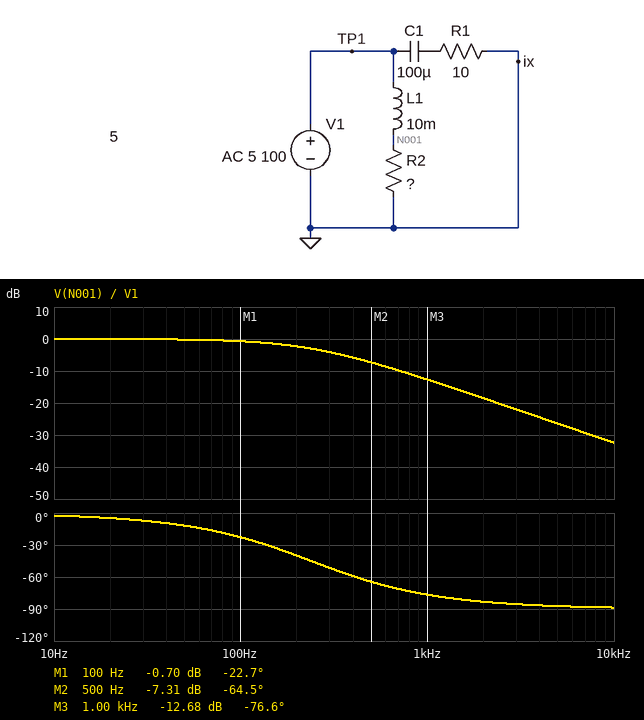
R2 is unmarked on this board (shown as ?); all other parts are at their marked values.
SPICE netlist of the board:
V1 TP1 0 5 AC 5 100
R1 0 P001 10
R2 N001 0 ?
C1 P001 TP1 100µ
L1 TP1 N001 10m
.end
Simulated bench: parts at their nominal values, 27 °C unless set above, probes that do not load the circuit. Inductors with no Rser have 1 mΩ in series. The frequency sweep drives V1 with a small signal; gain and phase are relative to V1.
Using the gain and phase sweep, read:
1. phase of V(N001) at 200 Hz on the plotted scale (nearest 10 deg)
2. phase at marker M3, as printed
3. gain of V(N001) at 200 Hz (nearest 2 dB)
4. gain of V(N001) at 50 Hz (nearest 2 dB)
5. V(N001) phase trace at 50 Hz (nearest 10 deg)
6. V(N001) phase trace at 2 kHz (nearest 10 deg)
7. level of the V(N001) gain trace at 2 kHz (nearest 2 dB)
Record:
-40 deg
-76.6 deg
-2 dB
0 dB
-10 deg
-80 deg
-18 dB
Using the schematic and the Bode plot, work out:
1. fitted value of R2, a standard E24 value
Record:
15 Ω
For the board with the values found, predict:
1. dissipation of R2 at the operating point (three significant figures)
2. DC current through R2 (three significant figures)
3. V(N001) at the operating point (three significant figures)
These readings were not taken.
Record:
1.67 W
333 mA
5.00 V
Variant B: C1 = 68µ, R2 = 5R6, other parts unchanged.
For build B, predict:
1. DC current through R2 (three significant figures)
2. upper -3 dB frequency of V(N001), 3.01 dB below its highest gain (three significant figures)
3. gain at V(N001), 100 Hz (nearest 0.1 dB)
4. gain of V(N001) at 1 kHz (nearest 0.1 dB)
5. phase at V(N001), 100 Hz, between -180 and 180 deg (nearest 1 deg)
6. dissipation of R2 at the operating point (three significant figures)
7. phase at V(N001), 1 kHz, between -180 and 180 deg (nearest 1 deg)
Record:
893 mA
89.1 Hz
-3.5 dB
-21.0 dB
-48 deg
4.46 W
-85 deg
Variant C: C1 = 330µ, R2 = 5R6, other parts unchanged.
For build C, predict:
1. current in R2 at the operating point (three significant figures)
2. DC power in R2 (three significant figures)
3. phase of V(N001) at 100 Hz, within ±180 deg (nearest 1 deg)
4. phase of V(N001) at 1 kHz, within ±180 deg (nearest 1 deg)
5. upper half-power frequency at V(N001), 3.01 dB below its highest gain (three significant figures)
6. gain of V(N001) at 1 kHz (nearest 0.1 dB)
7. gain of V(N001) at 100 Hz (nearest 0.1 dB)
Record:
893 mA
4.46 W
-48 deg
-85 deg
89.1 Hz
-21.0 dB
-3.5 dB
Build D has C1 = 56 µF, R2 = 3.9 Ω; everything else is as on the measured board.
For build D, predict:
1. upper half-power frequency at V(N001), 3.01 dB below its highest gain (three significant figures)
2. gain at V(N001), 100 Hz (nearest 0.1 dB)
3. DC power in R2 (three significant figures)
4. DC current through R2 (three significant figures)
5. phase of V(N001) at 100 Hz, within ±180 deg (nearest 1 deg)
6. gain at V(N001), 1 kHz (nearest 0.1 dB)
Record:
62.1 Hz
-5.6 dB
6.41 W
1.28 A
-58 deg
-24.2 dB
